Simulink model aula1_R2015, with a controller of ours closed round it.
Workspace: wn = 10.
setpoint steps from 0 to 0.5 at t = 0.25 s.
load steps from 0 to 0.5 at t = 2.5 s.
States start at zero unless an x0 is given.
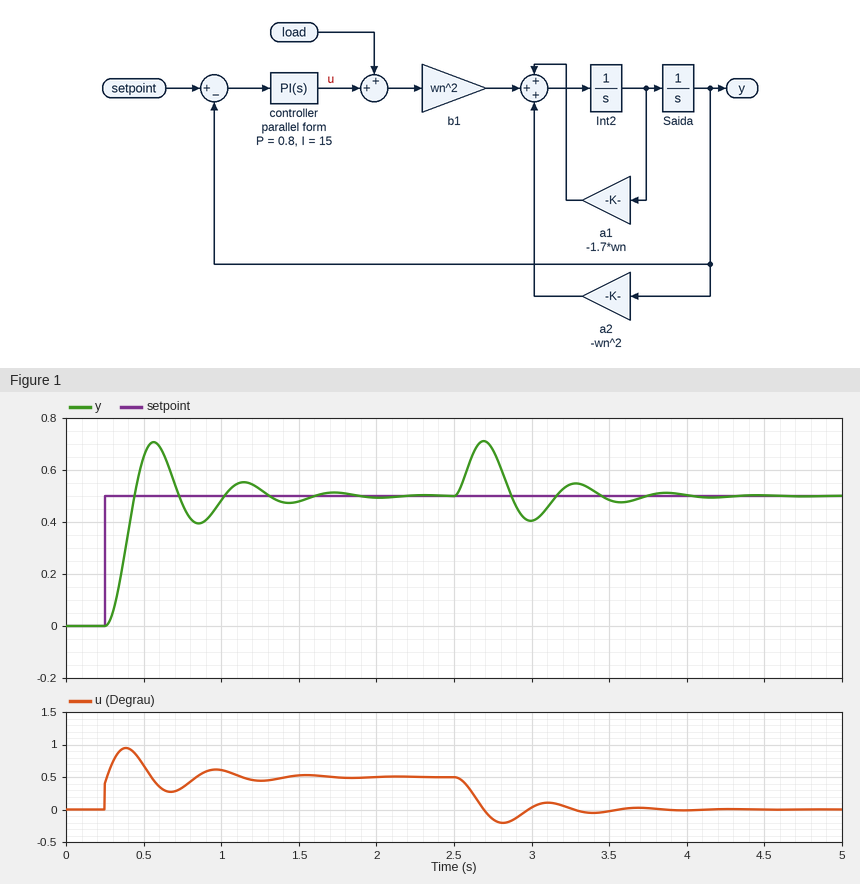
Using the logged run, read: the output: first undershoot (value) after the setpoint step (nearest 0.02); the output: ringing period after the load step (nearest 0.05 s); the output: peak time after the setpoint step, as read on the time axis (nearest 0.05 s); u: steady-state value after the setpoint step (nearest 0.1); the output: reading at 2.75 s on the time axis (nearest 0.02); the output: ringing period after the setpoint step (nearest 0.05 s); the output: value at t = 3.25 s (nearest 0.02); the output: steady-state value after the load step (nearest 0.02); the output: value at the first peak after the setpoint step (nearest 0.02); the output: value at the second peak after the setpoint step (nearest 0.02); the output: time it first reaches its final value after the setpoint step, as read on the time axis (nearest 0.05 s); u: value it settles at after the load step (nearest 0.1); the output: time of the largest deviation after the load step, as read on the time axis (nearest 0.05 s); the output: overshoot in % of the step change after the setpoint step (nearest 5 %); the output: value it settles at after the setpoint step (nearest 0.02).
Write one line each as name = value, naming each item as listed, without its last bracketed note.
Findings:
the output: first undershoot (value) after the setpoint step = 0.40
the output: ringing period after the load step = 0.60 s
the output: peak time after the setpoint step, as read on the time axis = 0.55 s
u: steady-state value after the setpoint step = 0.5
the output: reading at 2.75 s on the time axis = 0.68
the output: ringing period after the setpoint step = 0.60 s
the output: value at t = 3.25 s = 0.54
the output: steady-state value after the load step = 0.50
the output: value at the first peak after the setpoint step = 0.70
the output: value at the second peak after the setpoint step = 0.56
the output: time it first reaches its final value after the setpoint step, as read on the time axis = 0.45 s
u: value it settles at after the load step = 0.0
the output: time of the largest deviation after the load step, as read on the time axis = 2.70 s
the output: overshoot in % of the step change after the setpoint step = 40 %
the output: value it settles at after the setpoint step = 0.50
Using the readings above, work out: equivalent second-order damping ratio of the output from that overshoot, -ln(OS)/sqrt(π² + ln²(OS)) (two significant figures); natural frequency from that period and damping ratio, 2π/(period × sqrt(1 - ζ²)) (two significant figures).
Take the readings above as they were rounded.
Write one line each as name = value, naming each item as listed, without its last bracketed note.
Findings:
equivalent second-order damping ratio of the output from that overshoot, -ln(OS)/sqrt(π² + ln²(OS)) = 0.28
natural frequency from that period and damping ratio, 2π/(period × sqrt(1 - ζ²)) = 11 rad/s
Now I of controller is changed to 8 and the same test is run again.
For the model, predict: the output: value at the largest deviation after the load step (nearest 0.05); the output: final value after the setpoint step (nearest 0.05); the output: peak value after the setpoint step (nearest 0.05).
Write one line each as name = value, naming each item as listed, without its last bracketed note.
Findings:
the output: value at the largest deviation after the load step = 0.75
the output: final value after the setpoint step = 0.50
the output: peak value after the setpoint step = 0.55
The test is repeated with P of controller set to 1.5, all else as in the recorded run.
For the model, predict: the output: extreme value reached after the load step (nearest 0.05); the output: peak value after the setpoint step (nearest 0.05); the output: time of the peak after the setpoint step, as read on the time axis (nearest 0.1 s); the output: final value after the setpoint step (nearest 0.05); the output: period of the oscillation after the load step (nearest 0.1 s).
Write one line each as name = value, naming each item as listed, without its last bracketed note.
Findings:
the output: extreme value reached after the load step = 0.70
the output: peak value after the setpoint step = 0.65
the output: time of the peak after the setpoint step, as read on the time axis = 0.5 s
the output: final value after the setpoint step = 0.50
the output: period of the oscillation after the load step = 0.5 s
